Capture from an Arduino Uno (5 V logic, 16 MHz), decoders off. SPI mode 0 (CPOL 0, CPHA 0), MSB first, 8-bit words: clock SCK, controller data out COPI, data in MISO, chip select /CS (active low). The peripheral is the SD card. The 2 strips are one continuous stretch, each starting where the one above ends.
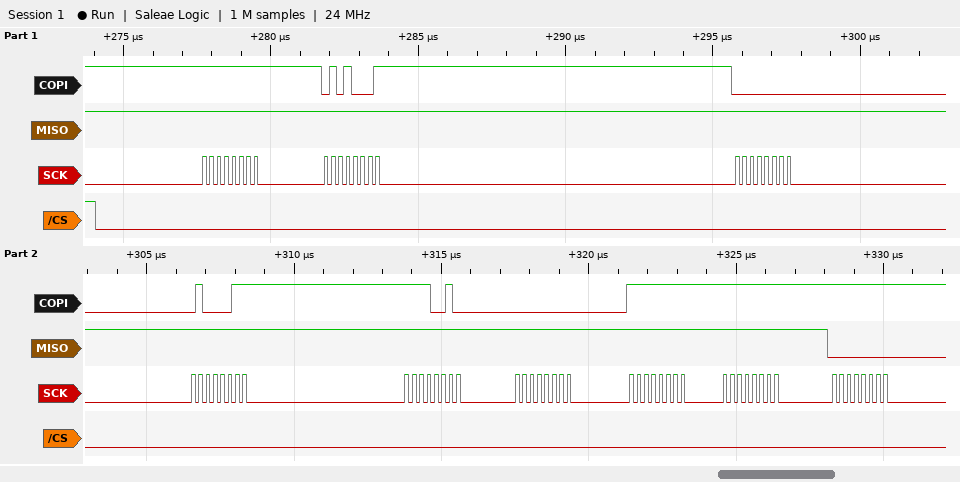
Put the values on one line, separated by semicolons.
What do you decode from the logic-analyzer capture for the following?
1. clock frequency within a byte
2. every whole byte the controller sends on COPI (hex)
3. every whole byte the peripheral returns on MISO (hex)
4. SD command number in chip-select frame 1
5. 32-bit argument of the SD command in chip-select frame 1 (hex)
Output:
4 MHz; 0xFF 0x51 0x00 0x43 0xF2 0x00 0xFF 0xFF 0xFF; 0xFF 0xFF 0xFF 0xFF 0xFF 0xFF 0xFF 0xFF 0x00; CMD17; 0x0043F200
